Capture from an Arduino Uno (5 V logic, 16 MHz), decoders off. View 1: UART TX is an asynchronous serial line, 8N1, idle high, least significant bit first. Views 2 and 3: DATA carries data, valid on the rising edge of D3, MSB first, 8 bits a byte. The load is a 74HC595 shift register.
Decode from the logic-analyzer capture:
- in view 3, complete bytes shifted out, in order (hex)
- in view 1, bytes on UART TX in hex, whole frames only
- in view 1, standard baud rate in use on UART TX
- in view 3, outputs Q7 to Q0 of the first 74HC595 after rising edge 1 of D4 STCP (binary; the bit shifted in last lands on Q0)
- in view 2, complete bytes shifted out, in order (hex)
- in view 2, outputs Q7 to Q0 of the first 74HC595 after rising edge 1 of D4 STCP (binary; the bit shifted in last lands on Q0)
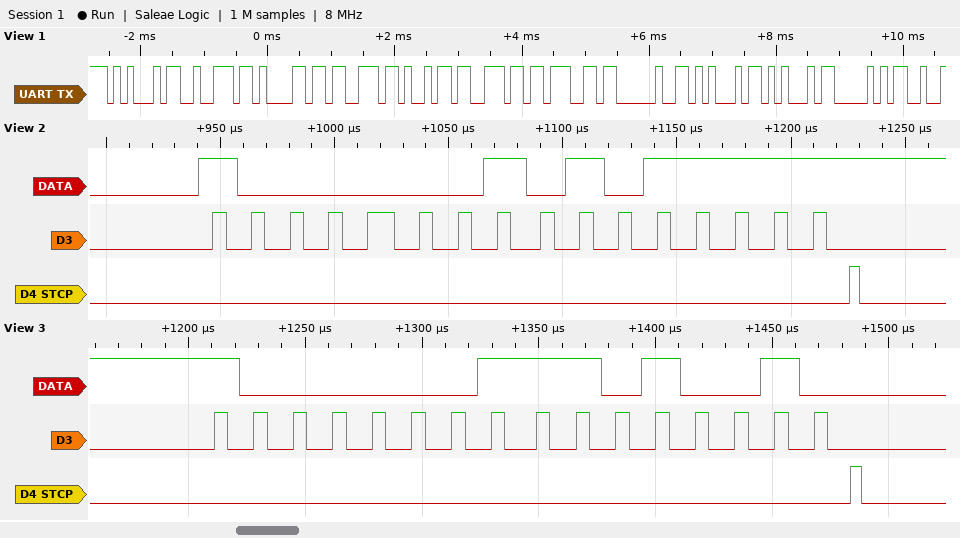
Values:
81 D2
45 72 61 73 69 6E 67 20 45 45 50
9600 baud
11010010
81 5F
01011111
